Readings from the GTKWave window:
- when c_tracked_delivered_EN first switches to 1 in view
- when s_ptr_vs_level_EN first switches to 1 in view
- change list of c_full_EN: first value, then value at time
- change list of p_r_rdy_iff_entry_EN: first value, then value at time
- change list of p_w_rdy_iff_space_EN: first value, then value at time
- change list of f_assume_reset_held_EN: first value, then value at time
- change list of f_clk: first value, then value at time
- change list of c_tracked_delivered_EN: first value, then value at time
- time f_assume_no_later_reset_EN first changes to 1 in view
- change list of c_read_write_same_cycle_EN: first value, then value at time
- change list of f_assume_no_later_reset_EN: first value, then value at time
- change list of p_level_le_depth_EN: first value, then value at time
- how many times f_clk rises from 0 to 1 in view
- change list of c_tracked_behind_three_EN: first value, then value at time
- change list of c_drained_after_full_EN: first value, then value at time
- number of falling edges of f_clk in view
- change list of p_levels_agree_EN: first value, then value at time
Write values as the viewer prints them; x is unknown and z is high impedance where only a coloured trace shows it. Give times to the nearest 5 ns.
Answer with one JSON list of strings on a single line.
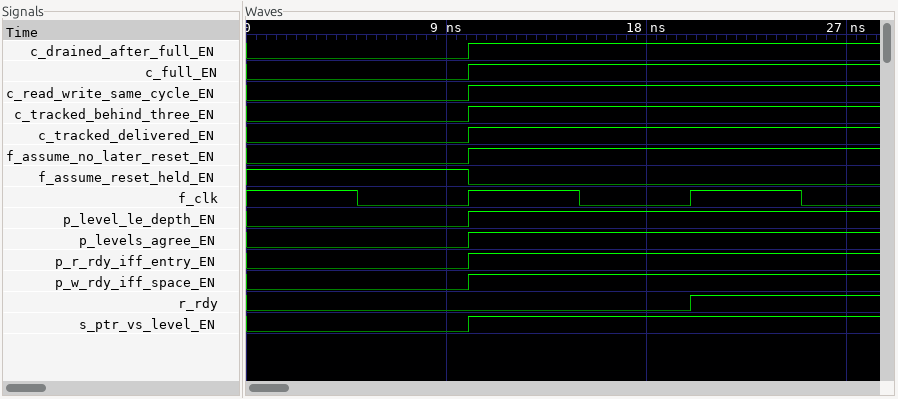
["10 ns", "10 ns", "0, 1 at 10 ns", "0, 1 at 10 ns", "0, 1 at 10 ns", "1, 0 at 10 ns", "1, 0 at 5 ns, 1 at 10 ns, 0 at 15 ns, 1 at 20 ns, 0 at 25 ns", "0, 1 at 10 ns", "10 ns", "0, 1 at 10 ns", "0, 1 at 10 ns", "0, 1 at 10 ns", "2", "0, 1 at 10 ns", "0, 1 at 10 ns", "3", "0, 1 at 10 ns"]
